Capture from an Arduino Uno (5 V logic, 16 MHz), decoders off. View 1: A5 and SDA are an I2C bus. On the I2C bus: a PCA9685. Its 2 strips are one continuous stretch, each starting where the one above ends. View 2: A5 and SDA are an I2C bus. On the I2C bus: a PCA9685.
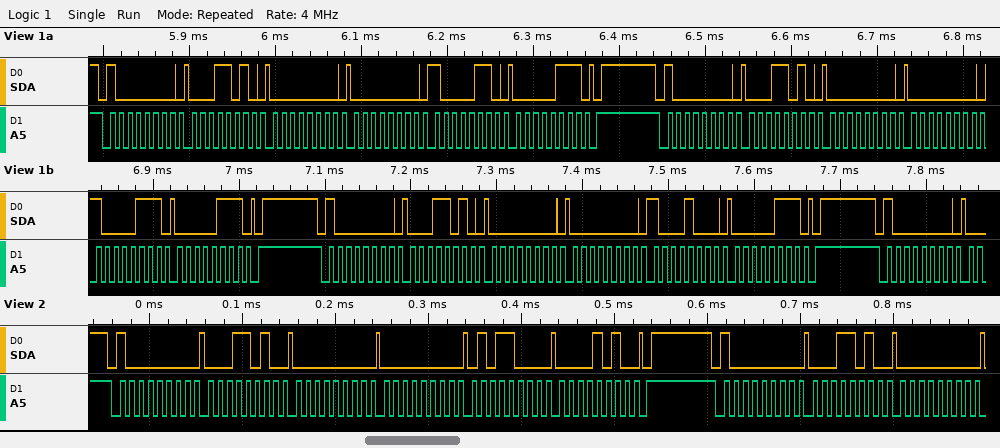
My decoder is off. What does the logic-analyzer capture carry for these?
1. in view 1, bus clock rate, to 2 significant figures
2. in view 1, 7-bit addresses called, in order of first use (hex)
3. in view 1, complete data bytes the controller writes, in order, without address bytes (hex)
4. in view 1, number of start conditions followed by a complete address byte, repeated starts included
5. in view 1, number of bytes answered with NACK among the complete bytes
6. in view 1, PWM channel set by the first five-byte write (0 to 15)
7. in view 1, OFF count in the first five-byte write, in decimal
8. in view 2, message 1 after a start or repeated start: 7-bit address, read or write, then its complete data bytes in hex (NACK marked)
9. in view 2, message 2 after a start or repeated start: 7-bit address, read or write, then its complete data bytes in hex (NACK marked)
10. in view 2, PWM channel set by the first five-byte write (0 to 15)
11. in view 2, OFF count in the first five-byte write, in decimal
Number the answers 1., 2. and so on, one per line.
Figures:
1. 100 kHz
2. 0x40
3. 1A 00 00 86 07 1A 00 00 87 07 1A 00 00 88 07
4. 4
5. 0
6. 5
7. 1926
8. 0x40 write: 1A 00 00 58 0A
9. 0x40 write: 1A 00
10. 5
11. 2648
